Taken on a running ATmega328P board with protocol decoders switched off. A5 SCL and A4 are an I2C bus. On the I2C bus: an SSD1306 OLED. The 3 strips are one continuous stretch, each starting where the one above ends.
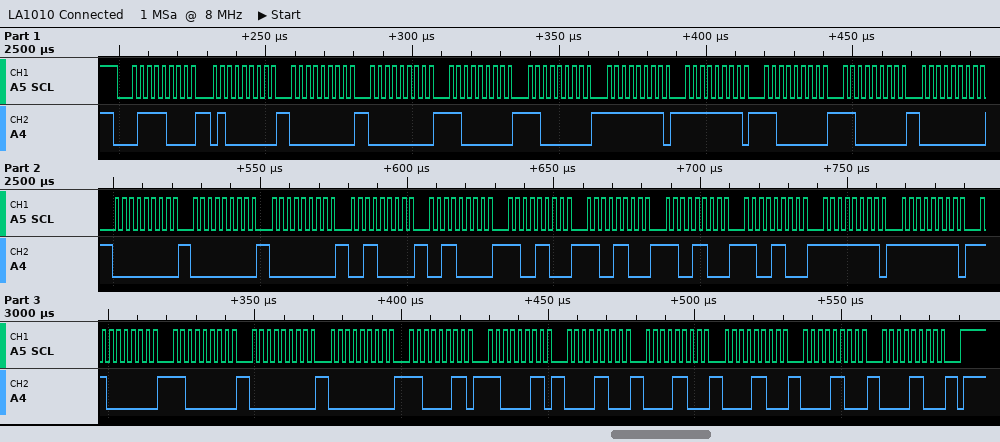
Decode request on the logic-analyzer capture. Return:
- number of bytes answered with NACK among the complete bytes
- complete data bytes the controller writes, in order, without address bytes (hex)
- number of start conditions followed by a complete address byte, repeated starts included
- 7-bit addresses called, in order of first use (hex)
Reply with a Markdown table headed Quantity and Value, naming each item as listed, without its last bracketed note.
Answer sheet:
| Quantity | Value |
|---|---|
| number of bytes answered with NACK among the complete bytes | 0 |
| complete data bytes the controller writes, in order, without address bytes | 40 00 00 C0 C0 FF FF C0 C0 00 00 00 00 30 30 CC CC CC CC FF FF C0 C0 00 00 C3 C3 0C 0C 0C 0C 0C |
| number of start conditions followed by a complete address byte, repeated starts included | 1 |
| 7-bit addresses called, in order of first use | 0x3C |
